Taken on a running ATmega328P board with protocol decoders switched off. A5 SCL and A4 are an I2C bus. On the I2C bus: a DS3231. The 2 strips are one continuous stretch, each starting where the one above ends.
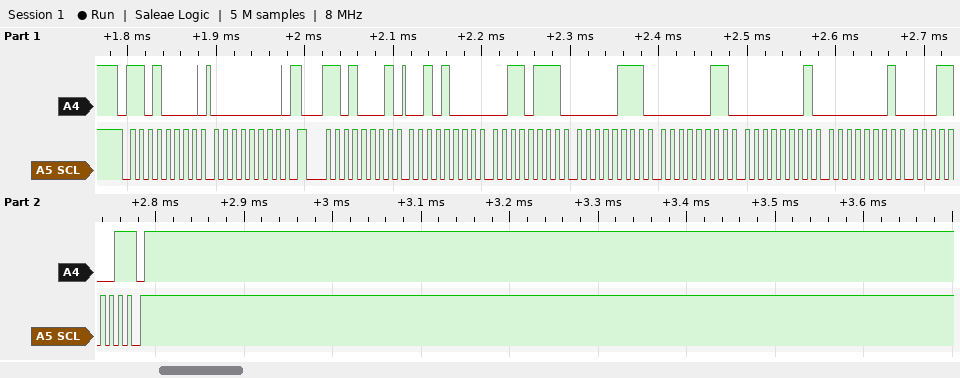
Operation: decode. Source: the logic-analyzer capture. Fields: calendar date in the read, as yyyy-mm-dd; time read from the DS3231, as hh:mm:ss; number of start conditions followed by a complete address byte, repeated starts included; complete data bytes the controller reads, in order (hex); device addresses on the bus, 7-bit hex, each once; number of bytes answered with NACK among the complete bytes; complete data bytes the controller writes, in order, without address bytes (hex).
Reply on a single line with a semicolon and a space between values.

2019-01-01; 07:37:28; 2; 28 37 07 03 01 01 19; 0x68; 1; 00
